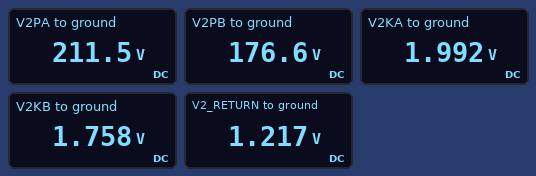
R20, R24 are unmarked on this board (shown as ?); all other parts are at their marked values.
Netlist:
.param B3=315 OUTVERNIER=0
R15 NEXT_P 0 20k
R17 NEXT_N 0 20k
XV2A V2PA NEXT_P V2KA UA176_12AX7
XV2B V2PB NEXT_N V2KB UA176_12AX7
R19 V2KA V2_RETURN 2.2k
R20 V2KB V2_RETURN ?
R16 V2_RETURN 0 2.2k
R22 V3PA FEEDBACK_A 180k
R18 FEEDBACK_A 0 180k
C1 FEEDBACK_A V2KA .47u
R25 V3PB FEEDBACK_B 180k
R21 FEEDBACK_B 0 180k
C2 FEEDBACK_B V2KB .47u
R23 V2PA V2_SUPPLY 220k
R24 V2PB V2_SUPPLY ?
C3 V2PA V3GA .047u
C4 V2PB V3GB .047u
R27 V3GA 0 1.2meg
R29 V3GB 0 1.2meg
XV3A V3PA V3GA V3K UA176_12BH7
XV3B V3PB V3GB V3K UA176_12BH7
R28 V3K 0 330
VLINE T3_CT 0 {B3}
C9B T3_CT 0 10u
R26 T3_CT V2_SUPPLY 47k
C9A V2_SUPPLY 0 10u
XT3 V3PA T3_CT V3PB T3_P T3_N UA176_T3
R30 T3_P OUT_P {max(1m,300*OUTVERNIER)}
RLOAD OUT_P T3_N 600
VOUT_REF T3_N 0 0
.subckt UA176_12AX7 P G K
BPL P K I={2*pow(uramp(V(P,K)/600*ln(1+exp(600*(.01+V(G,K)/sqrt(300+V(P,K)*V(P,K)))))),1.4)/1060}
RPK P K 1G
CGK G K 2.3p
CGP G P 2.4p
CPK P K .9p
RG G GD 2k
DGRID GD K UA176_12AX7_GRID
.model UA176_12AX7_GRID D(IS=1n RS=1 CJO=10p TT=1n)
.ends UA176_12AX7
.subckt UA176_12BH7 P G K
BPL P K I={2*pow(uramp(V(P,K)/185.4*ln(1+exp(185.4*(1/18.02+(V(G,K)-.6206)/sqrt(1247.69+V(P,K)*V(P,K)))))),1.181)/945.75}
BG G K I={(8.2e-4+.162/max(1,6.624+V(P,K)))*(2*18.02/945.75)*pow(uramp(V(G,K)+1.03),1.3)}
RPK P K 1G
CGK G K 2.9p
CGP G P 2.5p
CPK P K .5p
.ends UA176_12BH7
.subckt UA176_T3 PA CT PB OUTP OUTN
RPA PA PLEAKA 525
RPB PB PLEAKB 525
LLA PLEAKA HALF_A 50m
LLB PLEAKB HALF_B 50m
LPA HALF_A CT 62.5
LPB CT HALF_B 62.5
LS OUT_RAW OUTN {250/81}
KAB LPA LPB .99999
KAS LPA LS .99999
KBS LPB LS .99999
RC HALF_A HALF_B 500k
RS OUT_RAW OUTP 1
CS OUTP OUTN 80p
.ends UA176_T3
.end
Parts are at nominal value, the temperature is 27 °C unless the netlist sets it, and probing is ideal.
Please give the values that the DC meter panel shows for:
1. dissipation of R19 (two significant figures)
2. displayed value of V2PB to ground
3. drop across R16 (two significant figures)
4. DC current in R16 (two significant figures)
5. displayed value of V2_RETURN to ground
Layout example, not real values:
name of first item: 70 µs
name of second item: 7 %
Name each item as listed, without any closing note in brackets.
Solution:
dissipation of R19: 270 µW
displayed value of V2PB to ground: 176.6 V
drop across R16: 1.2 V
DC current in R16: 550 µA
displayed value of V2_RETURN to ground: 1.217 V
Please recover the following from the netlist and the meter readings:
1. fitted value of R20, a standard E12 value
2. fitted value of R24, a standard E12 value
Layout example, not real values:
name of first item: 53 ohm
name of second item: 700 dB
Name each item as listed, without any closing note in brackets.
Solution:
fitted value of R20, a standard E12 value: 2.7 kΩ
fitted value of R24, a standard E12 value: 560 kΩ
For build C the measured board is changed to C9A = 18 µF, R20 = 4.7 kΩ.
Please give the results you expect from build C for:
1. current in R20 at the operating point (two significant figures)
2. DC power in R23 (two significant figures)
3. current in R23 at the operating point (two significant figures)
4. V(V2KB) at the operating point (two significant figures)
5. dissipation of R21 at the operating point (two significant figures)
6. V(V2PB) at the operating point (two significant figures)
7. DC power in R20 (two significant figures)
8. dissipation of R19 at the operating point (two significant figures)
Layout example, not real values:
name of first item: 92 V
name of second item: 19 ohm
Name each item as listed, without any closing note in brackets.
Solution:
current in R20 at the operating point: 170 µA
DC power in R23: 29 mW
current in R23 at the operating point: 360 µA
V(V2KB) at the operating point: 2.0 V
dissipation of R21 at the operating point: 130 mW
V(V2PB) at the operating point: 190 V
DC power in R20: 140 µW
dissipation of R19 at the operating point: 290 µW
